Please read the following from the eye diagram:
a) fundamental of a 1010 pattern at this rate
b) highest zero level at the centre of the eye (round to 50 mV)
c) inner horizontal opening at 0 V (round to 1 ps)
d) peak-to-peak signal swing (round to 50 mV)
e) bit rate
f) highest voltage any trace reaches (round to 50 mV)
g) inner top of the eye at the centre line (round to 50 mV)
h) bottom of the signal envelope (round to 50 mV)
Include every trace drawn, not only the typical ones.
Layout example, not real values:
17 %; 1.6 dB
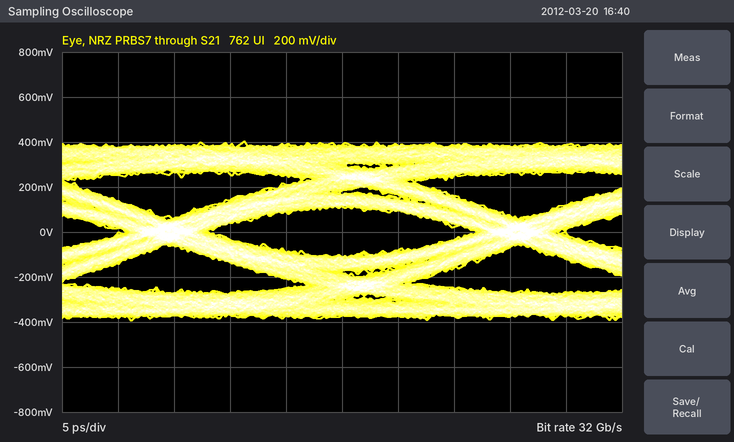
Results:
16 GHz; -100 mV; 24 ps; 800 mV; 32 Gb/s; 400 mV; 100 mV; -400 mV
